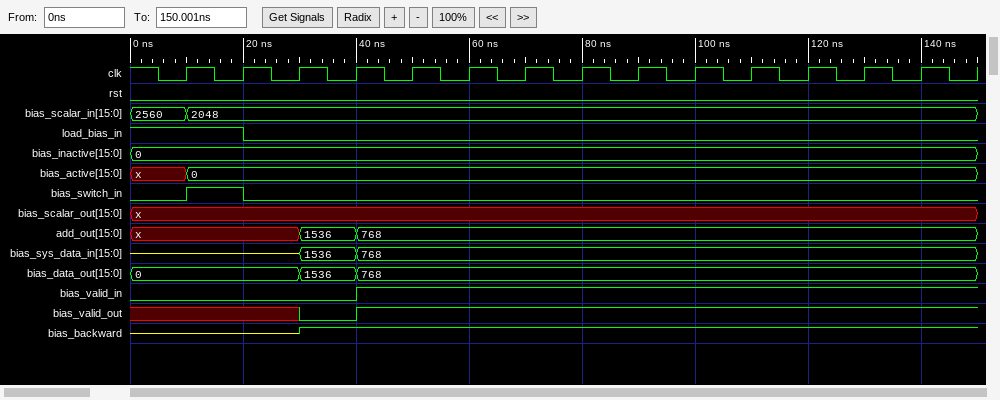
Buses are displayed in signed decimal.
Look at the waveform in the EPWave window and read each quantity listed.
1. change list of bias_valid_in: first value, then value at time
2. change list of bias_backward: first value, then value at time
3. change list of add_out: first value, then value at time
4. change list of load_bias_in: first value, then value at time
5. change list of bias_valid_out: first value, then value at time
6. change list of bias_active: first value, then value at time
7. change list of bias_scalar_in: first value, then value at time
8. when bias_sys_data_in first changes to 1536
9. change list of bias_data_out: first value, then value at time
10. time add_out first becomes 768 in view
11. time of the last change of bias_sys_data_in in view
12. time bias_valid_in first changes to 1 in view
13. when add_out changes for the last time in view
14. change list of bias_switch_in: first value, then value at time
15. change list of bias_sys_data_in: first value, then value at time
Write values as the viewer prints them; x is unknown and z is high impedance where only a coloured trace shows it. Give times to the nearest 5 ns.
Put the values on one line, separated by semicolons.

0, 1 at 40 ns; z, 1 at 30 ns; x, 1536 at 30 ns, 768 at 40 ns; 1, 0 at 20 ns; x, 0 at 30 ns, 1 at 40 ns; x, 0 at 10 ns; 2560, 2048 at 10 ns; 30 ns; 0, 1536 at 30 ns, 768 at 40 ns; 40 ns; 40 ns; 40 ns; 40 ns; 0, 1 at 10 ns, 0 at 20 ns; z, 1536 at 30 ns, 768 at 40 ns
